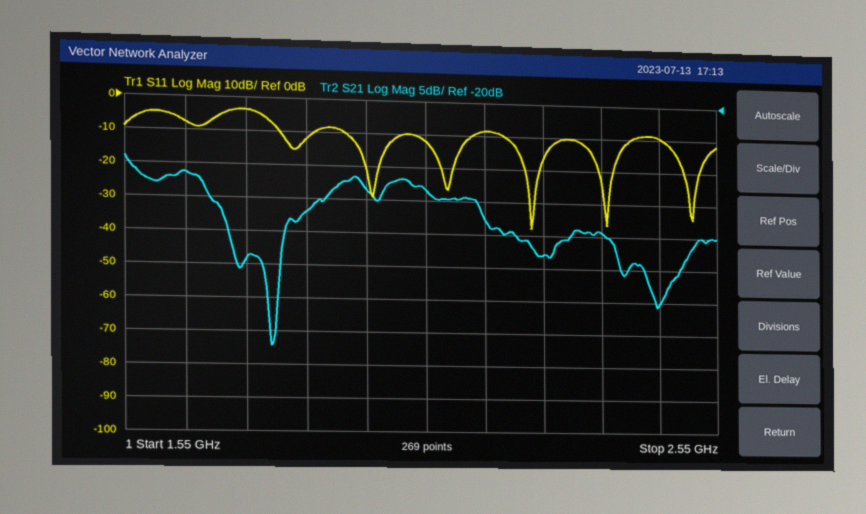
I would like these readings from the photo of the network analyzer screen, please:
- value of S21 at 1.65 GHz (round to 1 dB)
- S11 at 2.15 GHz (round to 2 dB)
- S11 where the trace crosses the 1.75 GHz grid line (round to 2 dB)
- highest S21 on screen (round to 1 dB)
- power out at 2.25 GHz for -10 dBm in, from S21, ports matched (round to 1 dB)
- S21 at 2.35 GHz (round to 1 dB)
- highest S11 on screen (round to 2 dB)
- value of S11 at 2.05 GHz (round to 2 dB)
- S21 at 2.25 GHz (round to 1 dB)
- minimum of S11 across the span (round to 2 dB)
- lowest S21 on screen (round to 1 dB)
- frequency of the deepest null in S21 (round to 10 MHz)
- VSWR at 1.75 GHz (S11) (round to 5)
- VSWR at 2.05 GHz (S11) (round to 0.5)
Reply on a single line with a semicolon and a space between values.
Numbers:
-31 dB; -8 dB; -4 dB; -29 dB; -53 dBm; -39 dB; -4 dB; -12 dB; -43 dB; -38 dB; -57 dB; 1.79 GHz; 5; 1.5
